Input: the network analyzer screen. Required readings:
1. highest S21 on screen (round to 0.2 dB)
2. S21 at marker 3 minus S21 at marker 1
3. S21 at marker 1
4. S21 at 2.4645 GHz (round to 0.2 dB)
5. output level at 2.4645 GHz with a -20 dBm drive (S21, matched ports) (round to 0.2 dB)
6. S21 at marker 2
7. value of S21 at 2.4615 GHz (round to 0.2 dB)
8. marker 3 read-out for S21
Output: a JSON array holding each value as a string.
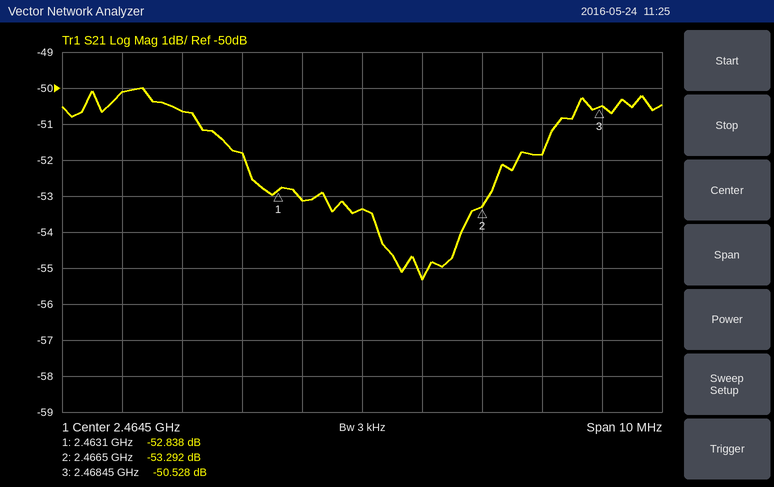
["-50.0 dB", "2.310 dB", "-52.838 dB", "-53.4 dB", "-73.4 dBm", "-53.292 dB", "-50.6 dB", "-50.528 dB"]
